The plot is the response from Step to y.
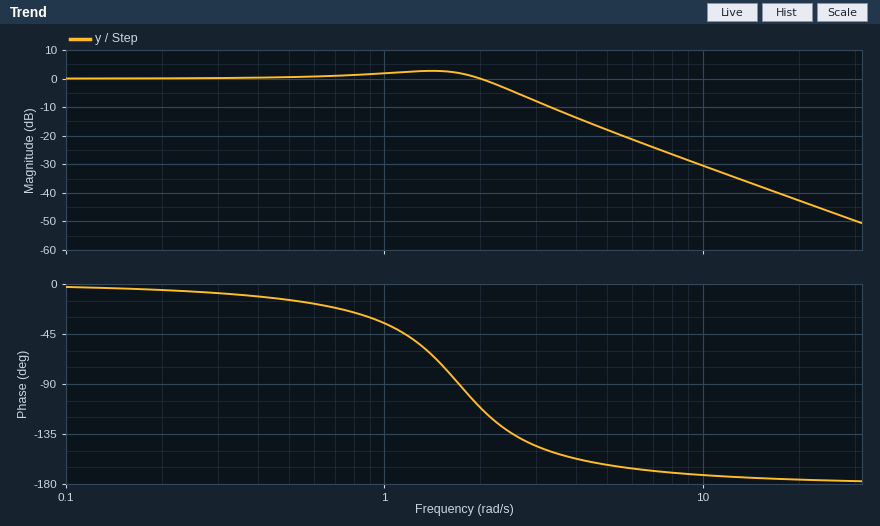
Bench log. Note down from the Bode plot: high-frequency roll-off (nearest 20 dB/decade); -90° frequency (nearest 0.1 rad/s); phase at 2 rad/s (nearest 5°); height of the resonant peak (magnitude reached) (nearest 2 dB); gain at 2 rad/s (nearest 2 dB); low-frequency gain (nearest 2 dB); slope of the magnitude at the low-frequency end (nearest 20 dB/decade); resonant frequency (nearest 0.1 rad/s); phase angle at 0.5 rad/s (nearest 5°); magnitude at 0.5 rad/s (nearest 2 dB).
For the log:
-40 dB/decade
1.7 rad/s
-110°
2 dB
0 dB
0 dB
0 dB/decade
1.4 rad/s
-15°
0 dB
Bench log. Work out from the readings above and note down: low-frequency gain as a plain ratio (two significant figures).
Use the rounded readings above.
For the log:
1.0
